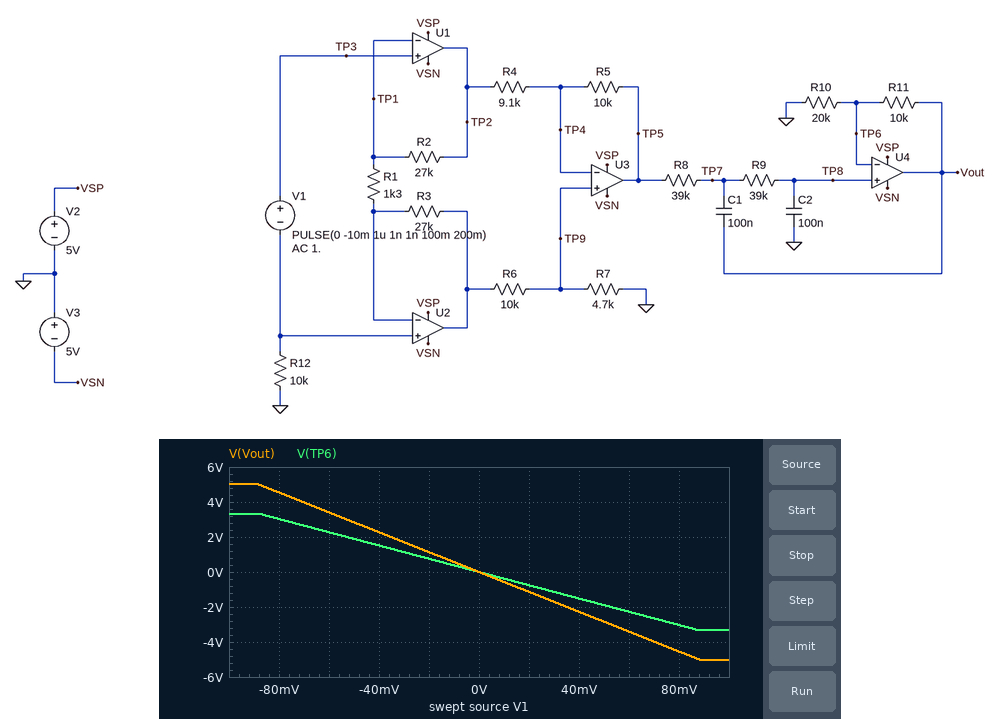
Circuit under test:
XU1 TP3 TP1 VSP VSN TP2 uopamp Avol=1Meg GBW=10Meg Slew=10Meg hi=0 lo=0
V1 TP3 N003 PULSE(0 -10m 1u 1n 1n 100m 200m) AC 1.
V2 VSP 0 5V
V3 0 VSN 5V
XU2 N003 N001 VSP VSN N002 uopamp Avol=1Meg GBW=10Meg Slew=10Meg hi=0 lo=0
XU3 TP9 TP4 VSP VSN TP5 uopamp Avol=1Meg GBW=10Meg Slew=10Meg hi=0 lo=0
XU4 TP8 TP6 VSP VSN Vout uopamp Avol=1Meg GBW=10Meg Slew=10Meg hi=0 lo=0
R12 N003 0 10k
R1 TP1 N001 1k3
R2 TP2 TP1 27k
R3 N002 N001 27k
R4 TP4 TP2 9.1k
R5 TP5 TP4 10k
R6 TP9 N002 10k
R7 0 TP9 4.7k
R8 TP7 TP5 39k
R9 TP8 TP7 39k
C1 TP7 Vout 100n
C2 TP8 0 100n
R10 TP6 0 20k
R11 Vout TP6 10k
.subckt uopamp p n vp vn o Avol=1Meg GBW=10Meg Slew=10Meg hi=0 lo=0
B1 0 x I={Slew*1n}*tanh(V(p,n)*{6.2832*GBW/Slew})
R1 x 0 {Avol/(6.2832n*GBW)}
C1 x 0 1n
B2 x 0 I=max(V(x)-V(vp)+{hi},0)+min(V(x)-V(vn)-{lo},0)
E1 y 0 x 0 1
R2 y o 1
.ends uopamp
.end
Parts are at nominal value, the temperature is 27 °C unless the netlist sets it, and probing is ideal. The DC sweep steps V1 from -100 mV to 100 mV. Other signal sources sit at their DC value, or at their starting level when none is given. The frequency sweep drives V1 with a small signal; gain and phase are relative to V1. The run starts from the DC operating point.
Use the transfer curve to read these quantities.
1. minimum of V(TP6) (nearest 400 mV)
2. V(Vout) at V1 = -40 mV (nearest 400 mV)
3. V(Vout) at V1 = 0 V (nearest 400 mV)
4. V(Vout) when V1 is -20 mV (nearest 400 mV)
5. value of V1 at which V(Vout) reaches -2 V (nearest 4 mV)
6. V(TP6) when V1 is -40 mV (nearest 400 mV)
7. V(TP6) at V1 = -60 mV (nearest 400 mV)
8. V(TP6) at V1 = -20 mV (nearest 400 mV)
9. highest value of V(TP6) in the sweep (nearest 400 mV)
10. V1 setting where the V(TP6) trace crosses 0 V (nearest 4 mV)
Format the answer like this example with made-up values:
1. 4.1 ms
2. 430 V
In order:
1. -3.2 V
2. 2.4 V
3. 0 V
4. 1.2 V
5. 36 mV
6. 1.6 V
7. 2.4 V
8. 800 mV
9. 3.2 V
10. 0 V
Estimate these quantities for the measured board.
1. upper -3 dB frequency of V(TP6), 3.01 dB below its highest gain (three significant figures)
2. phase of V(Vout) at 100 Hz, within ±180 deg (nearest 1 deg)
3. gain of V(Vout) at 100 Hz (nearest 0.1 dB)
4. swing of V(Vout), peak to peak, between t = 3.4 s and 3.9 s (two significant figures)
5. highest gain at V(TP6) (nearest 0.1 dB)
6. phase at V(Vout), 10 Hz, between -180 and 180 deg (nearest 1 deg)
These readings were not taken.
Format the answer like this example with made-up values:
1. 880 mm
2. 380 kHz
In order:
1. 38.3 Hz
2. 36 deg
3. 19.2 dB
4. 600 mV
5. 31.6 dB
6. 159 deg
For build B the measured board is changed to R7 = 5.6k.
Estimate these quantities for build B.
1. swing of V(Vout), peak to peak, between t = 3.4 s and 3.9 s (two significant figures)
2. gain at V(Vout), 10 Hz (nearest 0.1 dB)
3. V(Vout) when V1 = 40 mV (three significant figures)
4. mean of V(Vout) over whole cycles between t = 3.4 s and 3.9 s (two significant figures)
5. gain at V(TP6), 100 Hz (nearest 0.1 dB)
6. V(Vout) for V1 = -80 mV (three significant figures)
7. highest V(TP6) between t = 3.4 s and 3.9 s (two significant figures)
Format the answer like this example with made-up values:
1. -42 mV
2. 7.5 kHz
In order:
1. 630 mV
2. 35.4 dB
3. -2.37 V
4. 300 mV
5. 16.1 dB
6. 4.75 V
7. 410 mV
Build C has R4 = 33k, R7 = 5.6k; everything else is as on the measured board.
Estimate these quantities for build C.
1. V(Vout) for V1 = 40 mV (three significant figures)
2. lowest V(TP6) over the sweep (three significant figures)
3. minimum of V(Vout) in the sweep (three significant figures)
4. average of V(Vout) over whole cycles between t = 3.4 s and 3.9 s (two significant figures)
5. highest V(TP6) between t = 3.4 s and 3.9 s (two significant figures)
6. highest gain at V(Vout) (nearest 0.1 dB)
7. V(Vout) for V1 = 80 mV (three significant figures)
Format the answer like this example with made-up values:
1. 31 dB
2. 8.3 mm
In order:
1. -979 mV
2. -1.63 V
3. -2.45 V
4. 120 mV
5. 170 mV
6. 27.8 dB
7. -1.96 V
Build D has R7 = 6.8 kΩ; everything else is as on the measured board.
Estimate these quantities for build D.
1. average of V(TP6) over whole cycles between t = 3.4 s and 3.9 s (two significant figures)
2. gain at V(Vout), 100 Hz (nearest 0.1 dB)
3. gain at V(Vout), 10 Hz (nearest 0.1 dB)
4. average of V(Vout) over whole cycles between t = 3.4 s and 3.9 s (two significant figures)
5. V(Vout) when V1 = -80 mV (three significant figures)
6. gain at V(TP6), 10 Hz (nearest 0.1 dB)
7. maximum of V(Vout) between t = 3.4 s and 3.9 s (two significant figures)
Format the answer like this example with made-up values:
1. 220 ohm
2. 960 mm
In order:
1. 210 mV
2. 20.0 dB
3. 35.8 dB
4. 310 mV
5. 4.99 V
6. 32.3 dB
7. 640 mV
